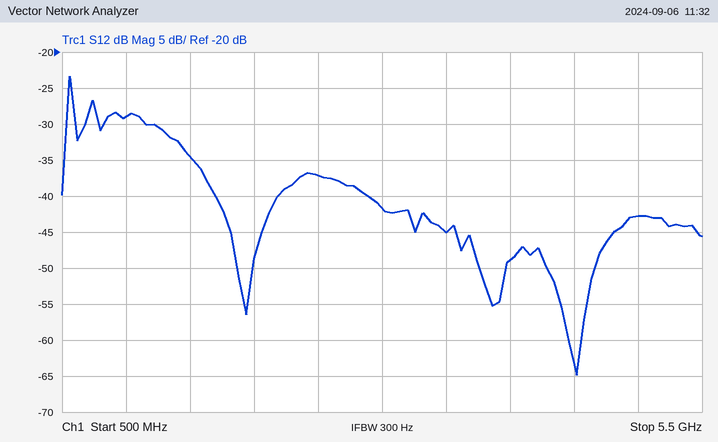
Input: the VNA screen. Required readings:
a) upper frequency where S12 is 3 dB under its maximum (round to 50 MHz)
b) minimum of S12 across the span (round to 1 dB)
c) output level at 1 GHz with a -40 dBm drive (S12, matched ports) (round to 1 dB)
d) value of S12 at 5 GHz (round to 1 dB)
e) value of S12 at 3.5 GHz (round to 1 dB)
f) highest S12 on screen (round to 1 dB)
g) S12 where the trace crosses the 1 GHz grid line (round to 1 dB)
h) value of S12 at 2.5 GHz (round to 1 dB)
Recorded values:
600 MHz
-65 dB
-69 dBm
-43 dB
-45 dB
-23 dB
-29 dB
-37 dB
